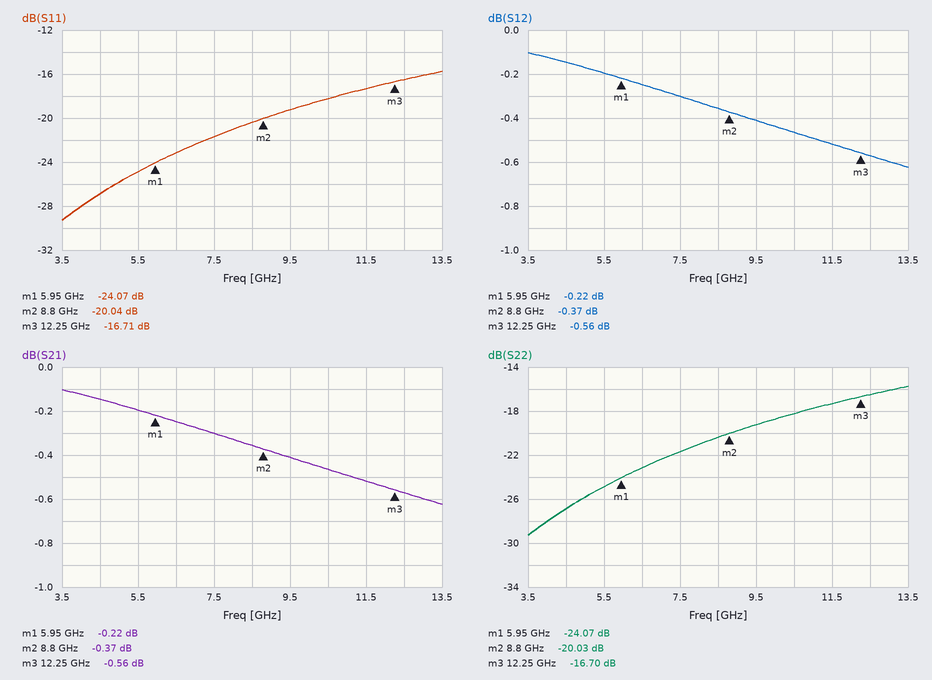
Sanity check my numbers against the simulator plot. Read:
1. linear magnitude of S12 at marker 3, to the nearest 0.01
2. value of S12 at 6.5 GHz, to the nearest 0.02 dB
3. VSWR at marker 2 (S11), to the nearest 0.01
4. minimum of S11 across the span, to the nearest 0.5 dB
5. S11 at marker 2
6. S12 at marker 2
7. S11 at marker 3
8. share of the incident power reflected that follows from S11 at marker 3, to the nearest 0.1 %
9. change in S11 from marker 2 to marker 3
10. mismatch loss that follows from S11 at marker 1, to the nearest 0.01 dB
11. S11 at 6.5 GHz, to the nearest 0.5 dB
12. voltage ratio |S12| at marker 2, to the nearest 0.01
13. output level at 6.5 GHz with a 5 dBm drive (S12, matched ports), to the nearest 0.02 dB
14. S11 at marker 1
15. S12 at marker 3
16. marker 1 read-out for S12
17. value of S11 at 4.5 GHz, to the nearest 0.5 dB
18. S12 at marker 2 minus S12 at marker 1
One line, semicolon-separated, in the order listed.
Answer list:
0.94; -0.24 dB; 1.22; -29.5 dB; -20.04 dB; -0.37 dB; -16.71 dB; 2.1 %; 3.33 dB; 0.02 dB; -23.0 dB; 0.96; 4.76 dBm; -24.07 dB; -0.56 dB; -0.22 dB; -27.0 dB; -0.15 dB
